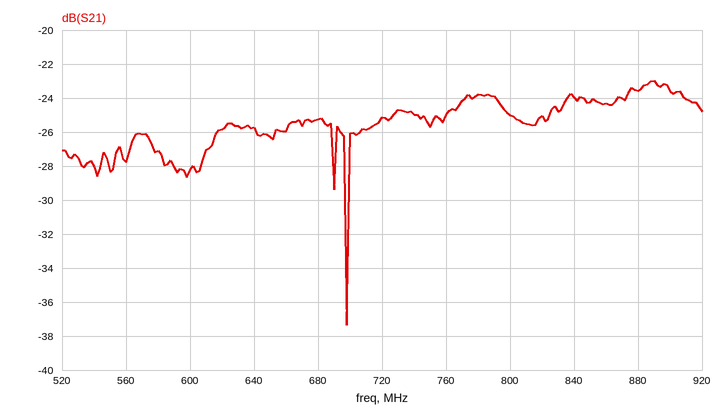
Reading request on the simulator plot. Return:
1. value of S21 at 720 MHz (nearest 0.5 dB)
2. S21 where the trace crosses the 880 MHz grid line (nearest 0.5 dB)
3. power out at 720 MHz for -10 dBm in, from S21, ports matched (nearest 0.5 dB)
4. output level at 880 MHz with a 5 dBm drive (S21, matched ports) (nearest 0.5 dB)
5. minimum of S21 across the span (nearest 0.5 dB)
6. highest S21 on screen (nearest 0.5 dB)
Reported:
-25.0 dB
-23.5 dB
-35.0 dBm
-18.5 dBm
-37.5 dB
-23.0 dB
